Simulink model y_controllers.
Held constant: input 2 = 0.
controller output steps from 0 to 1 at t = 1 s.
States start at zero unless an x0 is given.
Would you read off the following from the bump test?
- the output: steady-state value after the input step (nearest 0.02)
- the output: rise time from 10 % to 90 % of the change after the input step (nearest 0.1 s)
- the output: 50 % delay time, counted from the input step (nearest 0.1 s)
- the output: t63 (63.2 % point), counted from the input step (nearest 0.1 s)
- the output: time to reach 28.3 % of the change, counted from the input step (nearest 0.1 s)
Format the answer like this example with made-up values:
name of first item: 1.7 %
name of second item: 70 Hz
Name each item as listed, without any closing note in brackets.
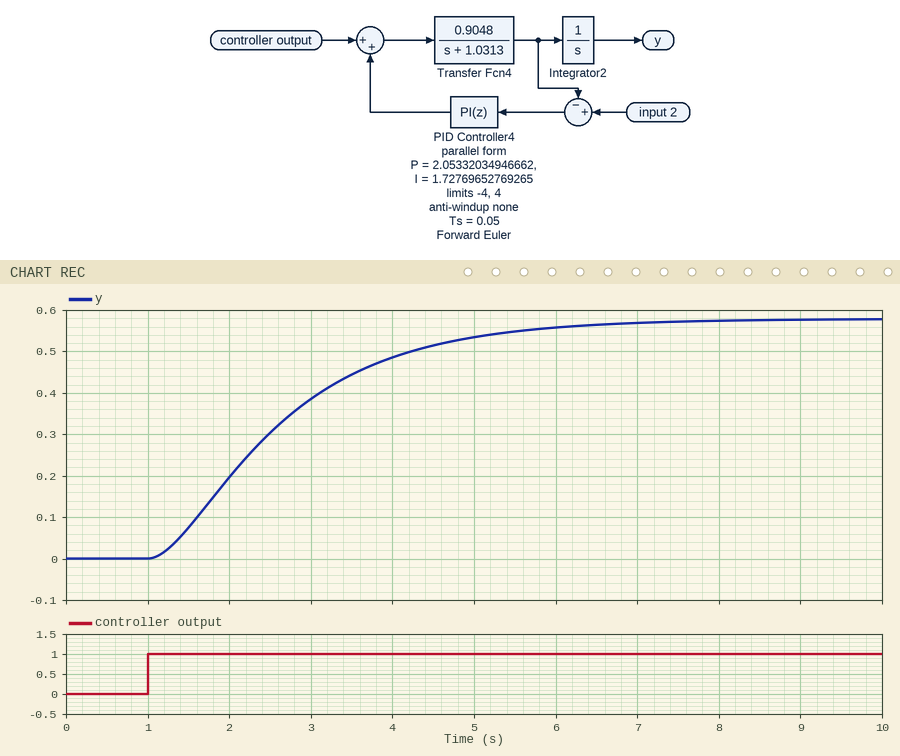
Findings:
the output: steady-state value after the input step: 0.58
the output: rise time from 10 % to 90 % of the change after the input step: 3.2 s
the output: 50 % delay time, counted from the input step: 1.4 s
the output: t63 (63.2 % point), counted from the input step: 1.9 s
the output: time to reach 28.3 % of the change, counted from the input step: 0.9 s
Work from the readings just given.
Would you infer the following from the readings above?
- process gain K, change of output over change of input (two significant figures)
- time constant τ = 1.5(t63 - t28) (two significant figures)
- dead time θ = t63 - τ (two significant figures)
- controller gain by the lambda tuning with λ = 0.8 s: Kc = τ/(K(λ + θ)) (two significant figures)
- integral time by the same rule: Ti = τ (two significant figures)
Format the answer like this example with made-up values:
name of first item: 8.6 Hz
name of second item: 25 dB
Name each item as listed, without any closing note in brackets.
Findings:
process gain K, change of output over change of input: 0.58
time constant τ = 1.5(t63 - t28): 1.5 s
dead time θ = t63 - τ: 0.40 s
controller gain by the lambda tuning with λ = 0.8 s: Kc = τ/(K(λ + θ)): 2.2
integral time by the same rule: Ti = τ: 1.5 s
